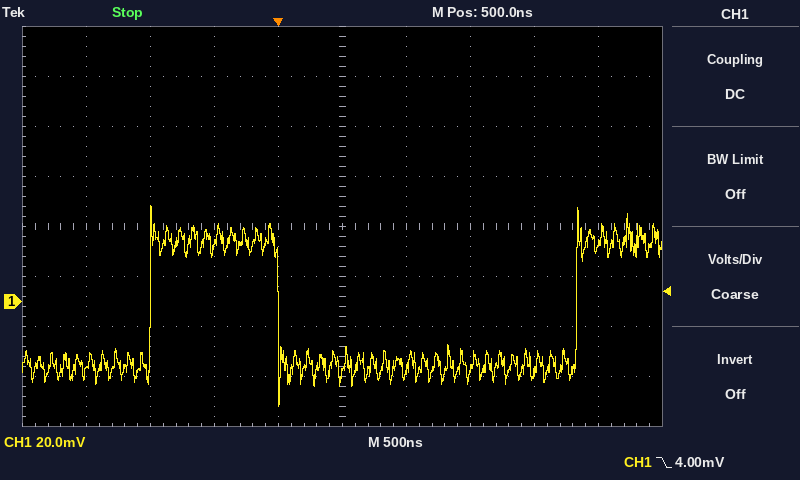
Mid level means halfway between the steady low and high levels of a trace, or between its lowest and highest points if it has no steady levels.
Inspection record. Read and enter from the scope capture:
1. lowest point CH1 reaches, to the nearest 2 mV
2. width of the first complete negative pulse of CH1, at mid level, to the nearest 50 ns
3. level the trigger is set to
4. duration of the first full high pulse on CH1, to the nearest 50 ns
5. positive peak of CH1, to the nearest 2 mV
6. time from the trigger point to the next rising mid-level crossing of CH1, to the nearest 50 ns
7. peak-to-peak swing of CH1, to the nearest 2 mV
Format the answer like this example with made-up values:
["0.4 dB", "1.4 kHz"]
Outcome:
["-42 mV", "2.35 µs", "4.00 mV", "1.00 µs", "38 mV", "2.35 µs", "80 mV"]
